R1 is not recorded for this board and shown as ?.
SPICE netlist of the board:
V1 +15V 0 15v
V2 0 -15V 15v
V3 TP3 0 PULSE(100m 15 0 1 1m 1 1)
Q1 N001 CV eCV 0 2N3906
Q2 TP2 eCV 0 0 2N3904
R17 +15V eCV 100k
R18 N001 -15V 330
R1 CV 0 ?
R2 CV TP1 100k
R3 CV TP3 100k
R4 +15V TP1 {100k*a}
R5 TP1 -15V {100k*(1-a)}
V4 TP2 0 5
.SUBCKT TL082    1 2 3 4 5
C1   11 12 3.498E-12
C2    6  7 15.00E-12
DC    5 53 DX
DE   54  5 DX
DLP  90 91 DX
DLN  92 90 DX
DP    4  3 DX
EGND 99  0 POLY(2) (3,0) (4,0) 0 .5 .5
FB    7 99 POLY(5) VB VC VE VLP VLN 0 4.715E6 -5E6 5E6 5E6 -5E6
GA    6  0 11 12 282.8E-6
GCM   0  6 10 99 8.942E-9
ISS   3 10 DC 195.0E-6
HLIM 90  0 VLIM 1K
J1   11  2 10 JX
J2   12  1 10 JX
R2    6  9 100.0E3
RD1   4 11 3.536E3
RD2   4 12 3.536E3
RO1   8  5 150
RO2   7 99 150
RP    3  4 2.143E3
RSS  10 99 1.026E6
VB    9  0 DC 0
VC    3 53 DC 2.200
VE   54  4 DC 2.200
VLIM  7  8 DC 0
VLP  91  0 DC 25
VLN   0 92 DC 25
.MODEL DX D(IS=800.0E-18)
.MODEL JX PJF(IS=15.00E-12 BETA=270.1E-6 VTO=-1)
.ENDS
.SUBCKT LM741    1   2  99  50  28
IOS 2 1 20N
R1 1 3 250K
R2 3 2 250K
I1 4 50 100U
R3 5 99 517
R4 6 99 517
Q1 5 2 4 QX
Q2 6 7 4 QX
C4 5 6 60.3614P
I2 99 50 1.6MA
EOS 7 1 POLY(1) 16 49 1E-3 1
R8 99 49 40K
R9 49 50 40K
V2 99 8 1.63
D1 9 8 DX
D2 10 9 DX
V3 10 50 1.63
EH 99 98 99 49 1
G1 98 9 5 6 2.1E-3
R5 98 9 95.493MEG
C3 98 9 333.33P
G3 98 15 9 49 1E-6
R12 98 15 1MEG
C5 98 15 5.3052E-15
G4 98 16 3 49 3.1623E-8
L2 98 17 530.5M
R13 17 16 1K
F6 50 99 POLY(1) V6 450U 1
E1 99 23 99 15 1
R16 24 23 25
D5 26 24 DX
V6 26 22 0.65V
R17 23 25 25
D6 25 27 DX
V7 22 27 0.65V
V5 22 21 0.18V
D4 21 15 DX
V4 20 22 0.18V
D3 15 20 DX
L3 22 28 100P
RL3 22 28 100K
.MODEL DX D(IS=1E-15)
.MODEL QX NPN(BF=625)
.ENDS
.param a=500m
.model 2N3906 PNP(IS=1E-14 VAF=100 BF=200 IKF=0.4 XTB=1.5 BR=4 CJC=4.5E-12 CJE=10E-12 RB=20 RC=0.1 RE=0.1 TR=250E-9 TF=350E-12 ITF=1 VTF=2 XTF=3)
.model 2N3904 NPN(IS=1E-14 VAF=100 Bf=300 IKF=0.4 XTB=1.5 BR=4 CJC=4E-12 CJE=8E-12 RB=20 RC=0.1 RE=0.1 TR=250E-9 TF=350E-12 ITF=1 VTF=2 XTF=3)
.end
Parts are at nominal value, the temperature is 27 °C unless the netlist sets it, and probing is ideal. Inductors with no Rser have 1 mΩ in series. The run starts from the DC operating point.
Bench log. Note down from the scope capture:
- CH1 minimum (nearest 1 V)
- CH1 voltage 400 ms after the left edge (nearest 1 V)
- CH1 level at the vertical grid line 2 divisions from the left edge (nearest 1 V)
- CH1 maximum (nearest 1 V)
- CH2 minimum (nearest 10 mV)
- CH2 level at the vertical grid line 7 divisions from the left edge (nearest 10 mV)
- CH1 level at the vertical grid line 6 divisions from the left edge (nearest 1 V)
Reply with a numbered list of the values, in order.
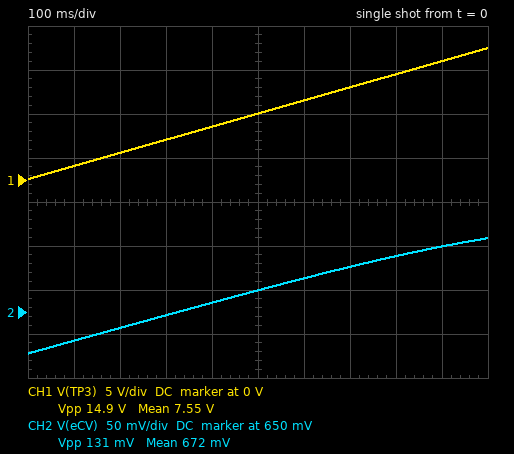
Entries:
1. 0 V
2. 6 V
3. 3 V
4. 15 V
5. 600 mV
6. 700 mV
7. 9 V
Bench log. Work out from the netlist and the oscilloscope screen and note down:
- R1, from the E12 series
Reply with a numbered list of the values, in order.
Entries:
1. 1 kΩ
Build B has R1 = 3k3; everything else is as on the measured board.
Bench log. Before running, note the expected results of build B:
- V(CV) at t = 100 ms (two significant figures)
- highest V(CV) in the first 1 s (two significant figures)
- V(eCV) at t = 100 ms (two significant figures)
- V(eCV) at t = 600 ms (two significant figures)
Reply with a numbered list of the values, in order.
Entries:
1. 51 mV
2. 470 mV
3. 650 mV
4. 760 mV
